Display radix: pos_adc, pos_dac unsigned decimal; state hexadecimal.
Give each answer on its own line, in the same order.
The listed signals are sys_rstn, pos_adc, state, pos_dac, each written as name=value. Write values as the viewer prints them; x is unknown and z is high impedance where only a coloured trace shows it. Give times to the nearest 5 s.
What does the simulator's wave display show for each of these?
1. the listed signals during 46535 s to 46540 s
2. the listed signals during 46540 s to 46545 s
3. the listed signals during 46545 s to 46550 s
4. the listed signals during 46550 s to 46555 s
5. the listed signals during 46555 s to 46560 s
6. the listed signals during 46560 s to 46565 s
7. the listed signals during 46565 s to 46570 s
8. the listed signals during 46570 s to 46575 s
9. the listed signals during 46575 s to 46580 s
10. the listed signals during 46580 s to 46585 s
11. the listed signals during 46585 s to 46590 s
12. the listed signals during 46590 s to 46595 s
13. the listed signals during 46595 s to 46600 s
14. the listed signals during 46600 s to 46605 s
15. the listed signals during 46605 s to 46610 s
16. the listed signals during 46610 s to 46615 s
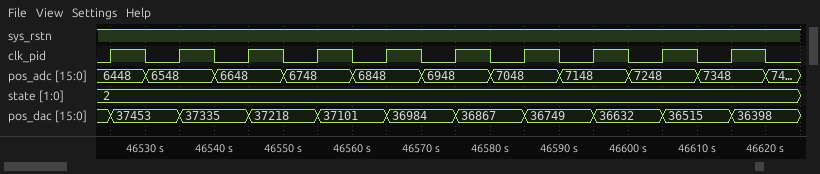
sys_rstn=1, pos_adc=6548, state=2, pos_dac=37335
sys_rstn=1, pos_adc=6648, state=2, pos_dac=37335
sys_rstn=1, pos_adc=6648, state=2, pos_dac=37218
sys_rstn=1, pos_adc=6748, state=2, pos_dac=37218
sys_rstn=1, pos_adc=6748, state=2, pos_dac=37101
sys_rstn=1, pos_adc=6848, state=2, pos_dac=37101
sys_rstn=1, pos_adc=6848, state=2, pos_dac=36984
sys_rstn=1, pos_adc=6948, state=2, pos_dac=36984
sys_rstn=1, pos_adc=6948, state=2, pos_dac=36867
sys_rstn=1, pos_adc=7048, state=2, pos_dac=36867
sys_rstn=1, pos_adc=7048, state=2, pos_dac=36749
sys_rstn=1, pos_adc=7148, state=2, pos_dac=36749
sys_rstn=1, pos_adc=7148, state=2, pos_dac=36632
sys_rstn=1, pos_adc=7248, state=2, pos_dac=36632
sys_rstn=1, pos_adc=7248, state=2, pos_dac=36515
sys_rstn=1, pos_adc=7348, state=2, pos_dac=36515
